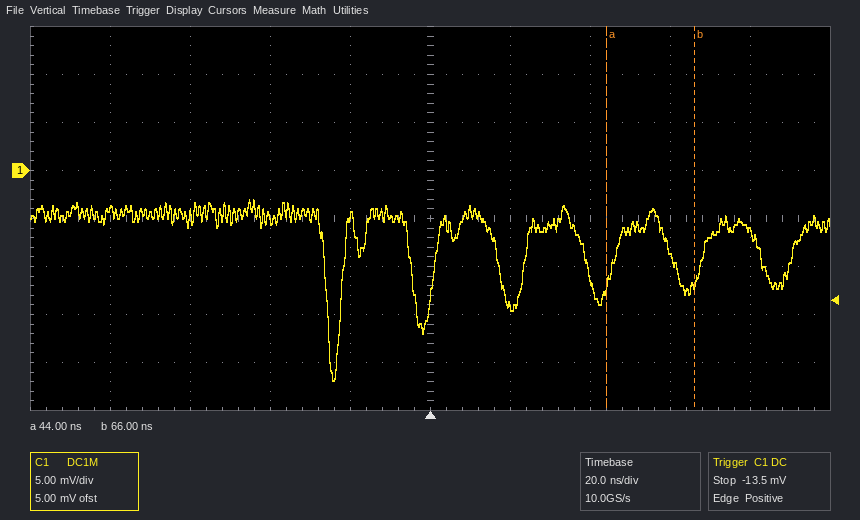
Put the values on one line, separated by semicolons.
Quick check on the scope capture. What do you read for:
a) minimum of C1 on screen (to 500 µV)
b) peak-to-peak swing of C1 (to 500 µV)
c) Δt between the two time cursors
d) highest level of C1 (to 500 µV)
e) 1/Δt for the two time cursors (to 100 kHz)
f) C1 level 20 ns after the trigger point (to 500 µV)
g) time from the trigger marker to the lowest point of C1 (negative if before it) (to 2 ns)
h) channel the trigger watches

-22.0 mV; 19.0 mV; 22 ns; -3.0 mV; 45.5 MHz; -14.0 mV; -24 ns; C1
